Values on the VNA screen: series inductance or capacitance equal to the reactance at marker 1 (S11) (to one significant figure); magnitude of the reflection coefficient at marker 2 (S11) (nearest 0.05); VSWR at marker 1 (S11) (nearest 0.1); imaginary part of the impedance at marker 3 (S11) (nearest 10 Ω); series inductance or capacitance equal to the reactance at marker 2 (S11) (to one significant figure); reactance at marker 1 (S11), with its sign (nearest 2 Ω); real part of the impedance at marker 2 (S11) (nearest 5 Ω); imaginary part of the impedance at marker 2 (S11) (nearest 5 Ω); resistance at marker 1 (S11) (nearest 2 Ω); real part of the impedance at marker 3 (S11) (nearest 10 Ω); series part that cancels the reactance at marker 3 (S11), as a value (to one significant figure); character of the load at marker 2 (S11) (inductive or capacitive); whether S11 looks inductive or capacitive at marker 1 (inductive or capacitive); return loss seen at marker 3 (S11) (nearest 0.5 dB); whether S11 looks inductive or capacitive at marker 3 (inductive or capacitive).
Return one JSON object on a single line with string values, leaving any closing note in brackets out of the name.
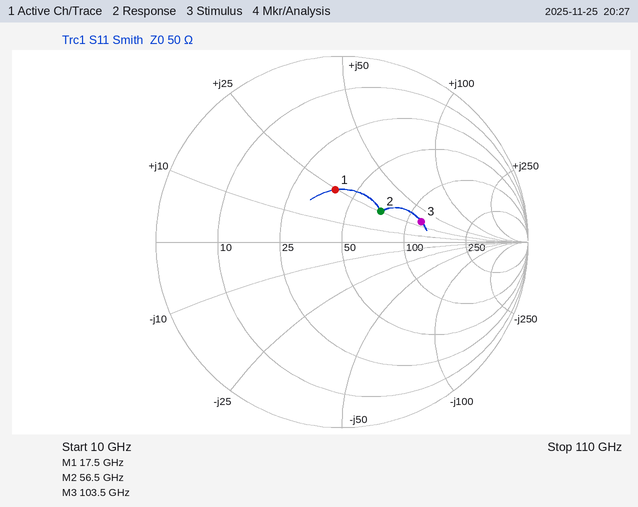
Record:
{"series inductance or capacitance equal to the reactance at marker 1 (S11)": "200 pH", "magnitude of the reflection coefficient at marker 2 (S11)": "0.25", "VSWR at marker 1 (S11)": "1.8", "imaginary part of the impedance at marker 3 (S11)": "+30 Ω", "series inductance or capacitance equal to the reactance at marker 2 (S11)": "70 pH", "reactance at marker 1 (S11), with its sign": "+24 Ω", "real part of the impedance at marker 2 (S11)": "70 Ω", "imaginary part of the impedance at marker 2 (S11)": "+25 Ω", "resistance at marker 1 (S11)": "40 Ω", "real part of the impedance at marker 3 (S11)": "120 Ω", "series part that cancels the reactance at marker 3 (S11), as a value": "50 fF", "character of the load at marker 2 (S11)": "inductive", "whether S11 looks inductive or capacitive at marker 1": "inductive", "return loss seen at marker 3 (S11)": "7.0 dB", "whether S11 looks inductive or capacitive at marker 3": "inductive"}
